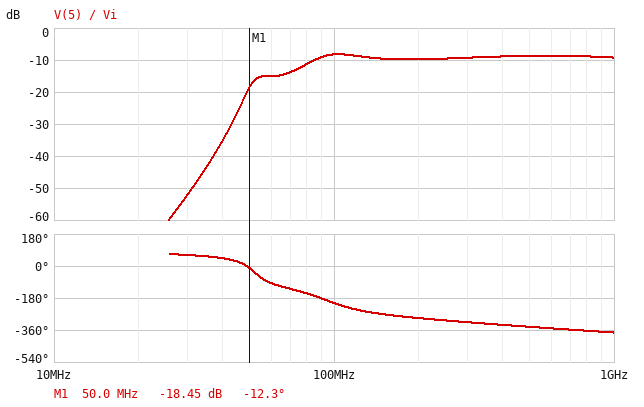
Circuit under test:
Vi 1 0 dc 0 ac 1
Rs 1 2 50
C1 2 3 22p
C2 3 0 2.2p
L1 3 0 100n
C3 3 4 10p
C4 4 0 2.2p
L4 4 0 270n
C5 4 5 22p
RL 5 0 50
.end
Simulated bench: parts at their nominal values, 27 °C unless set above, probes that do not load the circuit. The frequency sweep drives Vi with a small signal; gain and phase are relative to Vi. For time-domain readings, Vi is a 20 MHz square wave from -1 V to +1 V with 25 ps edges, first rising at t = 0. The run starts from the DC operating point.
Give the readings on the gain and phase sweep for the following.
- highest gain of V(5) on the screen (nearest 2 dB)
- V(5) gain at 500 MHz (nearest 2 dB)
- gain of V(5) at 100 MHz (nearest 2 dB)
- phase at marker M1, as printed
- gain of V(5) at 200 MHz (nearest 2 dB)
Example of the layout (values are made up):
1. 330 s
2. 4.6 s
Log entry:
1. -8 dB
2. -8 dB
3. -8 dB
4. -12.3 deg
5. -10 dB
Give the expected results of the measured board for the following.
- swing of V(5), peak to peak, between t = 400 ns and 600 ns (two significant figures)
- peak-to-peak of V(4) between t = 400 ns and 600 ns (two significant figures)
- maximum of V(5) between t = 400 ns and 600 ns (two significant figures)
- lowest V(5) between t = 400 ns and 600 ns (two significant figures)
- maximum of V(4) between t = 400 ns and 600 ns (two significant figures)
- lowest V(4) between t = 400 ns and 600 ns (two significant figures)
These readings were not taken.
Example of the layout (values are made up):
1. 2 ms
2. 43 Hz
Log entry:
1. 1.1 V
2. 1.3 V
3. 530 mV
4. -530 mV
5. 640 mV
6. -640 mV
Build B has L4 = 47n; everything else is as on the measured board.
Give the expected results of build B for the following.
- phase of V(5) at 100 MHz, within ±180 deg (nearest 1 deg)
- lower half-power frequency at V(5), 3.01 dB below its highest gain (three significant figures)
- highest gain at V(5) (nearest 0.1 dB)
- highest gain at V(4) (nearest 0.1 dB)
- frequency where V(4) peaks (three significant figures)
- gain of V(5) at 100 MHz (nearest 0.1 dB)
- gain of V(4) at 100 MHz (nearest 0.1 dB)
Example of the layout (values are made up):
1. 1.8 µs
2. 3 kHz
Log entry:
1. -114 deg
2. 109 MHz
3. -7.2 dB
4. -4.6 dB
5. 152 MHz
6. -10.9 dB
7. -6.0 dB
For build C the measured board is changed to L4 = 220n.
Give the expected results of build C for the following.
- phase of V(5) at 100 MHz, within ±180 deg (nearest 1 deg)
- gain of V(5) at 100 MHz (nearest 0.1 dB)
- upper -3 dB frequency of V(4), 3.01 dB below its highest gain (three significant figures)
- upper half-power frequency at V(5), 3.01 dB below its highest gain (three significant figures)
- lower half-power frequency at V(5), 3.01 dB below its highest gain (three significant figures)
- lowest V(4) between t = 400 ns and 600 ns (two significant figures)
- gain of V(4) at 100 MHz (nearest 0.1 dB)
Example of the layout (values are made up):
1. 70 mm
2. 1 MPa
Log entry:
1. 156 deg
2. -7.8 dB
3. 138 MHz
4. 1.61 GHz
5. 77.3 MHz
6. -520 mV
7. -2.9 dB
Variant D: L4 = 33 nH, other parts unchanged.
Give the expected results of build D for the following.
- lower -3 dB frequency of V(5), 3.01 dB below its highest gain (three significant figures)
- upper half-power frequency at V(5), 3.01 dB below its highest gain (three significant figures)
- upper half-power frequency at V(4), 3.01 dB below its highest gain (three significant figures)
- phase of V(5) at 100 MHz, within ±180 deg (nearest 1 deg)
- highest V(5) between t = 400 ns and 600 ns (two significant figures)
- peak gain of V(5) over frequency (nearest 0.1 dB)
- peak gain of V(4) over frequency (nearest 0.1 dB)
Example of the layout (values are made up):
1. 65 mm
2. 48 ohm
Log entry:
1. 150 MHz
2. 1.50 GHz
3. 1.04 GHz
4. -100 deg
5. 520 mV
6. -7.1 dB
7. -5.7 dB
